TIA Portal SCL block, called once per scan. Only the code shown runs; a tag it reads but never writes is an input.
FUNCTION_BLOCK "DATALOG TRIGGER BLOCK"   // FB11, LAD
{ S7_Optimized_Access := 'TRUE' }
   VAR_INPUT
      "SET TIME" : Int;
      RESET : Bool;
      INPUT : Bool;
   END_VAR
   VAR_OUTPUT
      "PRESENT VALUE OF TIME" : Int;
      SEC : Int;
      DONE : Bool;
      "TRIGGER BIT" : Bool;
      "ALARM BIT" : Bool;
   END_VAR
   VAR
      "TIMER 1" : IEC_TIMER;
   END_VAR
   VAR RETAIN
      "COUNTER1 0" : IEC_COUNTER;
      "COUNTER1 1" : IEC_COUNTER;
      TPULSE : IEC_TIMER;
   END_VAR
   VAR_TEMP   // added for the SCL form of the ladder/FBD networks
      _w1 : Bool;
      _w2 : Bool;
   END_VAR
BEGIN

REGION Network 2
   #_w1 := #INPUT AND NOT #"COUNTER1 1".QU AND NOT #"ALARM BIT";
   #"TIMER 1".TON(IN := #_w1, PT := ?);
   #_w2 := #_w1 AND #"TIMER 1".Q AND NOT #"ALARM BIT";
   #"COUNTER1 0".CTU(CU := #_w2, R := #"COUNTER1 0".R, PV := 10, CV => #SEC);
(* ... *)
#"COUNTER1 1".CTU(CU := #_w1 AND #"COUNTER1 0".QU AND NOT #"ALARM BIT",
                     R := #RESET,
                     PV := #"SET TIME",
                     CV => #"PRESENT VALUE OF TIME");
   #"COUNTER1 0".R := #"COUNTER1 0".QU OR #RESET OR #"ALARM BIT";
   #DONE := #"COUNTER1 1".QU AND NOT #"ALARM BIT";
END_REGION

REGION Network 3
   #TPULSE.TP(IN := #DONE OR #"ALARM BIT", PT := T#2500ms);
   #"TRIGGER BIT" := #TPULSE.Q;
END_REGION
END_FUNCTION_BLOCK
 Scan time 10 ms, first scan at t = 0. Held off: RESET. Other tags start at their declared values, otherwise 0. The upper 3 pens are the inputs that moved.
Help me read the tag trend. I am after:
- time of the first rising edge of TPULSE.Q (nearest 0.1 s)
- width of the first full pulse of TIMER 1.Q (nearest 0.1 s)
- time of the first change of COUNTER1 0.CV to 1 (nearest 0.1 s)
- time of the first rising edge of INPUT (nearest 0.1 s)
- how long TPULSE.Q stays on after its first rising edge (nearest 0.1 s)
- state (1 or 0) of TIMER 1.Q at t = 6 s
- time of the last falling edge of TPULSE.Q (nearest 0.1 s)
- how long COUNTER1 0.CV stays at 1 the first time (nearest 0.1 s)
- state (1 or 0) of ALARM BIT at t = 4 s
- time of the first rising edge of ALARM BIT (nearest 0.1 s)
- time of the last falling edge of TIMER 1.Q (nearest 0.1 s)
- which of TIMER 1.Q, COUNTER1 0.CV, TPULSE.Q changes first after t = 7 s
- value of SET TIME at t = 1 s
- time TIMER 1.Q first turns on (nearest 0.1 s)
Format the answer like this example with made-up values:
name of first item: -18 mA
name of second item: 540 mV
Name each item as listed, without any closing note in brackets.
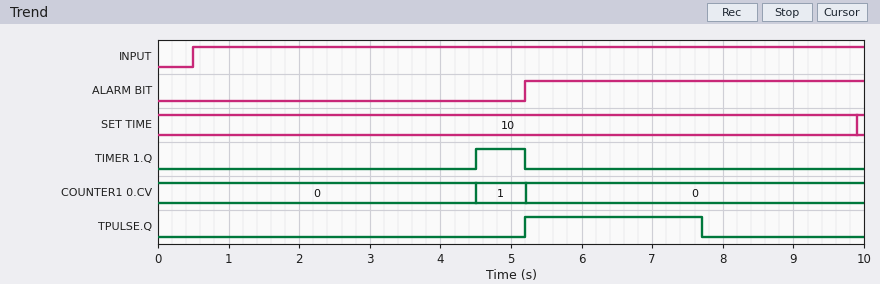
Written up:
time of the first rising edge of TPULSE.Q: 5.2 s
width of the first full pulse of TIMER 1.Q: 0.7 s
time of the first change of COUNTER1 0.CV to 1: 4.5 s
time of the first rising edge of INPUT: 0.5 s
how long TPULSE.Q stays on after its first rising edge: 2.5 s
state (1 or 0) of TIMER 1.Q at t = 6 s: 0
time of the last falling edge of TPULSE.Q: 7.7 s
how long COUNTER1 0.CV stays at 1 the first time: 0.7 s
state (1 or 0) of ALARM BIT at t = 4 s: 0
time of the first rising edge of ALARM BIT: 5.2 s
time of the last falling edge of TIMER 1.Q: 5.2 s
which of TIMER 1.Q, COUNTER1 0.CV, TPULSE.Q changes first after t = 7 s: TPULSE.Q
value of SET TIME at t = 1 s: 10
time TIMER 1.Q first turns on: 4.5 s
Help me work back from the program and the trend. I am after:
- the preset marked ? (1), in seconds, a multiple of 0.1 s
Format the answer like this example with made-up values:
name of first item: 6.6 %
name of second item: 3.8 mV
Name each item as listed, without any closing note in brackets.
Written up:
the preset marked ? (1), in seconds, a multiple of 0.1 s: 4.0 s
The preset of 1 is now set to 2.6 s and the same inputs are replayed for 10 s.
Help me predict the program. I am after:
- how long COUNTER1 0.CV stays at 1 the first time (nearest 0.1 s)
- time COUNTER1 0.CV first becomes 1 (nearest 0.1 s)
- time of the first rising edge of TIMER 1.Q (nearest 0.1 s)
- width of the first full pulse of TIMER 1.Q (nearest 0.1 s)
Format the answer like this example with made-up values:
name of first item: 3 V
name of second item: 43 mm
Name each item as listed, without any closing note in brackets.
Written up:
how long COUNTER1 0.CV stays at 1 the first time: 2.1 s
time COUNTER1 0.CV first becomes 1: 3.1 s
time of the first rising edge of TIMER 1.Q: 3.1 s
width of the first full pulse of TIMER 1.Q: 2.1 s
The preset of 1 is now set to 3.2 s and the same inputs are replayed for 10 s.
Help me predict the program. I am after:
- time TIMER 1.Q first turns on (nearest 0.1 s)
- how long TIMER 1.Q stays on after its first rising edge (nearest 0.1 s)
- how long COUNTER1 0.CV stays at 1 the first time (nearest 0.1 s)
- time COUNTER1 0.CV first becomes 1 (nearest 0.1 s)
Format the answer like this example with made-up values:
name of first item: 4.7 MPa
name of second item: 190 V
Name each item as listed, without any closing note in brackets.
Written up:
time TIMER 1.Q first turns on: 3.7 s
how long TIMER 1.Q stays on after its first rising edge: 1.5 s
how long COUNTER1 0.CV stays at 1 the first time: 1.5 s
time COUNTER1 0.CV first becomes 1: 3.7 s
